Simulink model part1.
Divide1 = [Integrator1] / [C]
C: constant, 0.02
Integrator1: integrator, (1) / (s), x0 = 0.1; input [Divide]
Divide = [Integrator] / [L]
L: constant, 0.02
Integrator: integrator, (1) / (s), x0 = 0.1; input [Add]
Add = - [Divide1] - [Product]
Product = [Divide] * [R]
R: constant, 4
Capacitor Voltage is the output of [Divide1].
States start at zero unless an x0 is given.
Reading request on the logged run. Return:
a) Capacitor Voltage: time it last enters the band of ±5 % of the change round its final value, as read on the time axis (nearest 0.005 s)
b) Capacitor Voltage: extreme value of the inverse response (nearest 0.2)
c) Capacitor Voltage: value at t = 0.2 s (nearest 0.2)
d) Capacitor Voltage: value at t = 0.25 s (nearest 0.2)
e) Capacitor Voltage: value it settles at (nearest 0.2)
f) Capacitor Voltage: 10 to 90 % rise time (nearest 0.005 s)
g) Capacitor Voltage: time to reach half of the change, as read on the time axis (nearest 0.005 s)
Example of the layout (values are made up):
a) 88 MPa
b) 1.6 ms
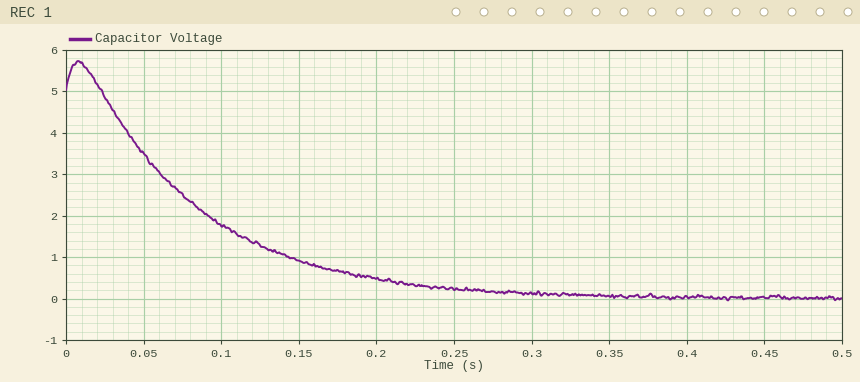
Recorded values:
a) 0.245 s
b) 5.8
c) 0.4
d) 0.2
e) 0.0
f) 0.165 s
g) 0.075 s
